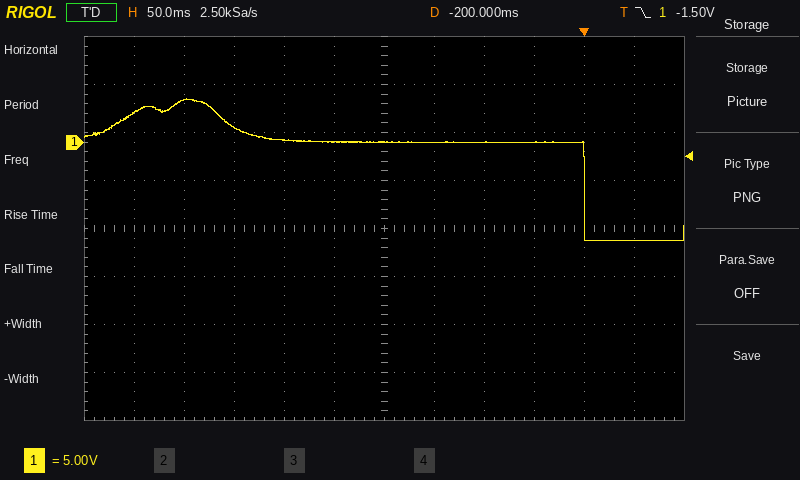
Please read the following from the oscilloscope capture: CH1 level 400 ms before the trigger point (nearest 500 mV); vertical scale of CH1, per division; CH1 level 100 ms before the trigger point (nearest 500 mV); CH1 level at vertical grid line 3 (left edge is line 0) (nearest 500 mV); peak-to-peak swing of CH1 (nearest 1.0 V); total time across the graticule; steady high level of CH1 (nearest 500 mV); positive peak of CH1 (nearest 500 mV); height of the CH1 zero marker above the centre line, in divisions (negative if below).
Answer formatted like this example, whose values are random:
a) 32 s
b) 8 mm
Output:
a) 4.5 V
b) 5 V
c) 0.0 V
d) 1.5 V
e) 15.0 V
f) 600 ms
g) 0.0 V
h) 4.5 V
i) +1.8 div
